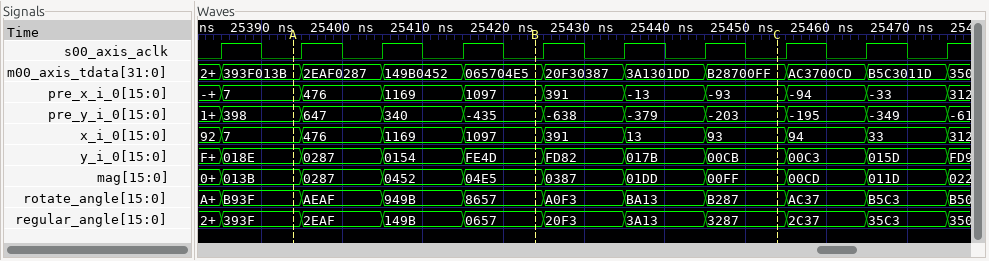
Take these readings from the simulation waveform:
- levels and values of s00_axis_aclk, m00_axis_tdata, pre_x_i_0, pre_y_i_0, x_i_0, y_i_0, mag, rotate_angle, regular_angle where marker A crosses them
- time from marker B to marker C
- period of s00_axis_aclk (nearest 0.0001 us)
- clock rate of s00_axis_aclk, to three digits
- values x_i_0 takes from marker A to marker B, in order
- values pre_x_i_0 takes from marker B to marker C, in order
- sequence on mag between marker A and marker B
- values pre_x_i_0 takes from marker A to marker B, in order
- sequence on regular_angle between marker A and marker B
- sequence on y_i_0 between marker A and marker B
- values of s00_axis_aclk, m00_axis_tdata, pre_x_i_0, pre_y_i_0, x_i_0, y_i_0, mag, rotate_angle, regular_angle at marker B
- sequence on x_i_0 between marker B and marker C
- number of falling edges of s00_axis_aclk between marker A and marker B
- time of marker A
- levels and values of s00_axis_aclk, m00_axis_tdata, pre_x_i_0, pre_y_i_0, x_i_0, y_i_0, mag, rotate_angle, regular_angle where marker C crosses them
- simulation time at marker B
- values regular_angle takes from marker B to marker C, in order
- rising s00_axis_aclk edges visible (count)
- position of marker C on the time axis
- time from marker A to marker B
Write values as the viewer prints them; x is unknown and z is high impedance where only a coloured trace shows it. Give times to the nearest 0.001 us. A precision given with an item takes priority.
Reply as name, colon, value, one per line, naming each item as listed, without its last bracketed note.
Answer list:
levels and values of s00_axis_aclk, m00_axis_tdata, pre_x_i_0, pre_y_i_0, x_i_0, y_i_0, mag, rotate_angle, regular_angle where marker A crosses them: s00_axis_aclk=0, m00_axis_tdata=393F013B, pre_x_i_0=7, pre_y_i_0=398, x_i_0=7, y_i_0=018E, mag=013B, rotate_angle=B93F, regular_angle=393F
time from marker B to marker C: 0.03 us
period of s00_axis_aclk: 0.01 us
clock rate of s00_axis_aclk, to three digits: 100 MHz
values x_i_0 takes from marker A to marker B, in order: 7, 476, 1169, 1097
values pre_x_i_0 takes from marker B to marker C, in order: 1097, 391, -13, -93
sequence on mag between marker A and marker B: 013B, 0287, 0452, 04E5
values pre_x_i_0 takes from marker A to marker B, in order: 7, 476, 1169, 1097
sequence on regular_angle between marker A and marker B: 393F, 2EAF, 149B, 0657
sequence on y_i_0 between marker A and marker B: 018E, 0287, 0154, FE4D
values of s00_axis_aclk, m00_axis_tdata, pre_x_i_0, pre_y_i_0, x_i_0, y_i_0, mag, rotate_angle, regular_angle at marker B: s00_axis_aclk=0, m00_axis_tdata=065704E5, pre_x_i_0=1097, pre_y_i_0=-435, x_i_0=1097, y_i_0=FE4D, mag=04E5, rotate_angle=8657, regular_angle=0657
sequence on x_i_0 between marker B and marker C: 1097, 391, 13, 93
number of falling edges of s00_axis_aclk between marker A and marker B: 3
time of marker A: 25.394 us
levels and values of s00_axis_aclk, m00_axis_tdata, pre_x_i_0, pre_y_i_0, x_i_0, y_i_0, mag, rotate_angle, regular_angle where marker C crosses them: s00_axis_aclk=0, m00_axis_tdata=B28700FF, pre_x_i_0=-93, pre_y_i_0=-203, x_i_0=93, y_i_0=00CB, mag=00FF, rotate_angle=B287, regular_angle=3287
simulation time at marker B: 25.424 us
values regular_angle takes from marker B to marker C, in order: 0657, 20F3, 3A13, 3287
rising s00_axis_aclk edges visible: 10
position of marker C on the time axis: 25.454 us
time from marker A to marker B: 0.03 us
